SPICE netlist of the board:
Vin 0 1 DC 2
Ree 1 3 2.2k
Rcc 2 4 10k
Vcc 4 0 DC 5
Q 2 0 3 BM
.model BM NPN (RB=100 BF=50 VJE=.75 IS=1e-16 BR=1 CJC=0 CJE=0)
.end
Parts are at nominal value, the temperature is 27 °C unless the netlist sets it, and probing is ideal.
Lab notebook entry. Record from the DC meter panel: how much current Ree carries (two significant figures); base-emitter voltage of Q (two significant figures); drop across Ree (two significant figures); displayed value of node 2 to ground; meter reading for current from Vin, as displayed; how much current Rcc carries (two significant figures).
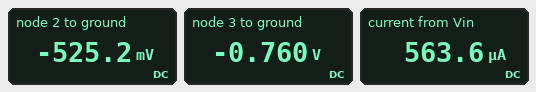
560 µA
760 mV
1.2 V
-525.2 mV
563.6 µA
550 µA
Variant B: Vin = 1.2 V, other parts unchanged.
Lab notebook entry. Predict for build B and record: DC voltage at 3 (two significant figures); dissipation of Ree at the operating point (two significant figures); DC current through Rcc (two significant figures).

-730 mV
99 µW
210 µA
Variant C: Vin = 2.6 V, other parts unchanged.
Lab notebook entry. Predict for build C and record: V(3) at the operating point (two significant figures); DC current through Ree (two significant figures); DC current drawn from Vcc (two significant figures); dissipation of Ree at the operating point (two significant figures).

-800 mV
820 µA
580 µA
1.5 mW
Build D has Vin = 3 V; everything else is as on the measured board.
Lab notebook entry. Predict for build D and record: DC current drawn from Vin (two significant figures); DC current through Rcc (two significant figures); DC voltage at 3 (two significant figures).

990 µA
580 µA
-820 mV
